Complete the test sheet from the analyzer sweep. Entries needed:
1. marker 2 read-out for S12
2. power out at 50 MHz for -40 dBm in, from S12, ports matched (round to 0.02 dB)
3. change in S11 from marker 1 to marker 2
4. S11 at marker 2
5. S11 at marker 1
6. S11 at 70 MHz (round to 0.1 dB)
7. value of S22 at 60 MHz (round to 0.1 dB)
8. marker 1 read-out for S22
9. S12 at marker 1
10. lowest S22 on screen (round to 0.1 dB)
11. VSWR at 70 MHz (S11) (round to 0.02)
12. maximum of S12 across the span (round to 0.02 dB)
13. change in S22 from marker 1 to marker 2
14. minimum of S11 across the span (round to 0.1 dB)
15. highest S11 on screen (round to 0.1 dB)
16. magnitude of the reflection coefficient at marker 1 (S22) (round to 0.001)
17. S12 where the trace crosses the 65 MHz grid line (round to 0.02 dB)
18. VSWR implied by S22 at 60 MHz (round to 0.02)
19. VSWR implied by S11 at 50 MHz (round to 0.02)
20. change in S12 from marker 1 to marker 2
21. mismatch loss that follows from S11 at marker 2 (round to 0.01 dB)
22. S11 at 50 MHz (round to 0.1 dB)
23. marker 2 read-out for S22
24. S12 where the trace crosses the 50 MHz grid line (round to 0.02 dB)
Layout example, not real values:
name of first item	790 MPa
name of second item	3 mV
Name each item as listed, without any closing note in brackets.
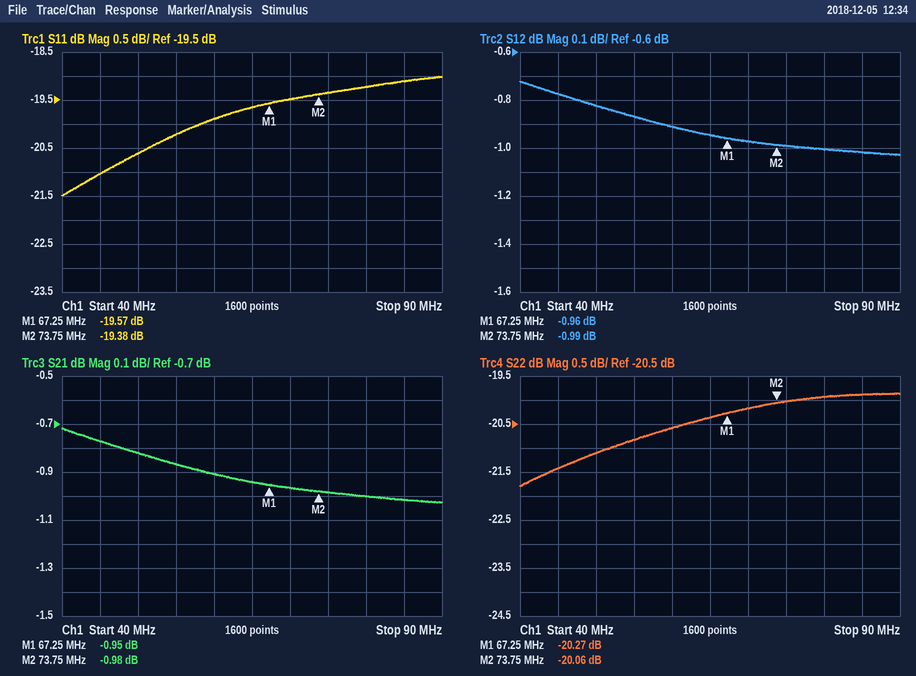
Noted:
marker 2 read-out for S12	-0.99 dB
power out at 50 MHz for -40 dBm in, from S12, ports matched	-40.82 dBm
change in S11 from marker 1 to marker 2	0.19 dB
S11 at marker 2	-19.38 dB
S11 at marker 1	-19.57 dB
S11 at 70 MHz	-19.5 dB
value of S22 at 60 MHz	-20.6 dB
marker 1 read-out for S22	-20.27 dB
S12 at marker 1	-0.96 dB
lowest S22 on screen	-21.8 dB
VSWR at 70 MHz (S11)	1.24
maximum of S12 across the span	-0.72 dB
change in S22 from marker 1 to marker 2	0.21 dB
minimum of S11 across the span	-21.5 dB
highest S11 on screen	-19.0 dB
magnitude of the reflection coefficient at marker 1 (S22)	0.097
S12 where the trace crosses the 65 MHz grid line	-0.94 dB
VSWR implied by S22 at 60 MHz	1.20
VSWR implied by S11 at 50 MHz	1.20
change in S12 from marker 1 to marker 2	-0.03 dB
mismatch loss that follows from S11 at marker 2	0.05 dB
S11 at 50 MHz	-20.6 dB
marker 2 read-out for S22	-20.06 dB
S12 where the trace crosses the 50 MHz grid line	-0.82 dB
